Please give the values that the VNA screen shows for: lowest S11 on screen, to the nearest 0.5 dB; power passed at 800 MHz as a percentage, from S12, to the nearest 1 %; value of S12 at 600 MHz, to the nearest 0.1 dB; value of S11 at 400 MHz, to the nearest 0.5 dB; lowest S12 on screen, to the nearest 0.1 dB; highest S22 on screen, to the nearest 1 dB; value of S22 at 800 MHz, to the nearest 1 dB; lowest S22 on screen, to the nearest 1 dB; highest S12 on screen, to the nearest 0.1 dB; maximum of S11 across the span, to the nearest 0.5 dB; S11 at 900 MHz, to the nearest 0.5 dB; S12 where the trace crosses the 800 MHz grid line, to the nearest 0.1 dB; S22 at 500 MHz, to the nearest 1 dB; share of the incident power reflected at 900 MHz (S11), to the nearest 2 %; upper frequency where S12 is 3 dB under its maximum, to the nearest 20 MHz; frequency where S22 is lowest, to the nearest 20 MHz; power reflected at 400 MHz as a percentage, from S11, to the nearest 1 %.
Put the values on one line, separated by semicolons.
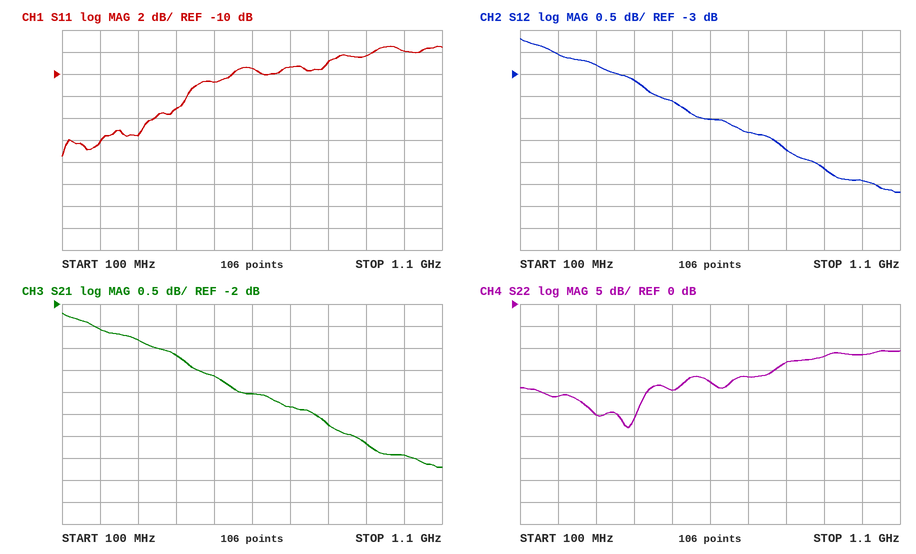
-17.5 dB; 34 %; -4.0 dB; -13.0 dB; -5.7 dB; -11 dB; -13 dB; -28 dB; -2.2 dB; -7.5 dB; -8.5 dB; -4.7 dB; -20 dB; 14 %; 900 MHz; 380 MHz; 5 %
